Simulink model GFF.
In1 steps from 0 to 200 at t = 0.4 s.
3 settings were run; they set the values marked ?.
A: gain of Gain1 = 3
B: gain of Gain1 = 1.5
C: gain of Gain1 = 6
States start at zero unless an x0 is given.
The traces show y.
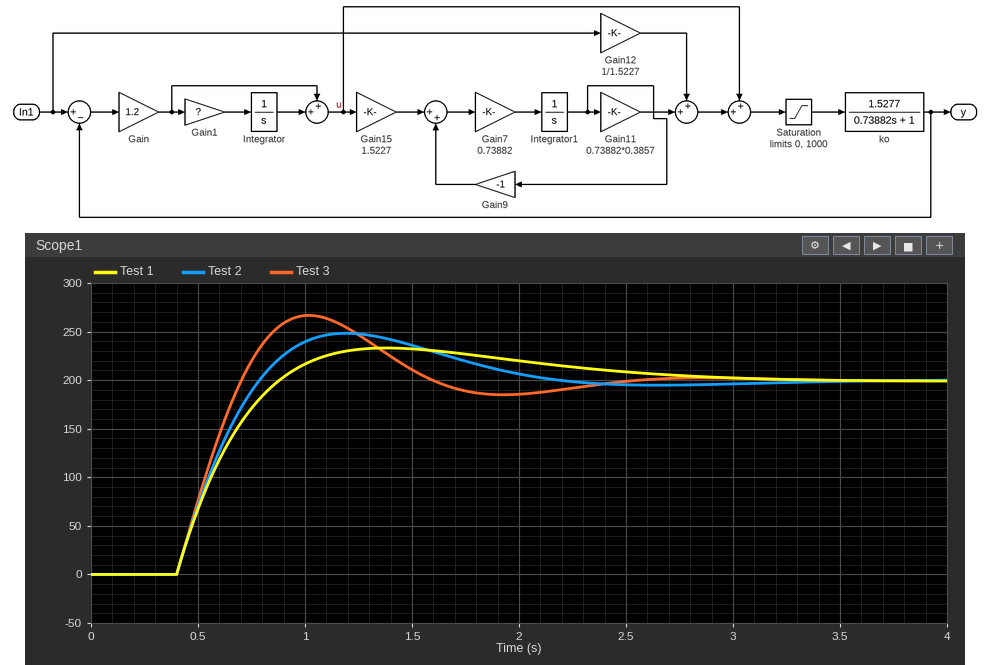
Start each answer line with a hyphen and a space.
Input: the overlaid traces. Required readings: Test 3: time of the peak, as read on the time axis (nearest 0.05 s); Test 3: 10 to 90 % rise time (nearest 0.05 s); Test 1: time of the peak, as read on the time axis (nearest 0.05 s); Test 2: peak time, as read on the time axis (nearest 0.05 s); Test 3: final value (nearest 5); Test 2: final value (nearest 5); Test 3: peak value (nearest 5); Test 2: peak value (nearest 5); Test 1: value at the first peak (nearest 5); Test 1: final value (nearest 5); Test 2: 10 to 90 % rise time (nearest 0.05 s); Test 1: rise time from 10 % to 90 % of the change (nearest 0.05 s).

- 1.00 s
- 0.25 s
- 1.40 s
- 1.20 s
- 200
- 200
- 265
- 250
- 235
- 200
- 0.30 s
- 0.35 s
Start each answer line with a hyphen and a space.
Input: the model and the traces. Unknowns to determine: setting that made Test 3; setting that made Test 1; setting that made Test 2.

- C
- B
- A
